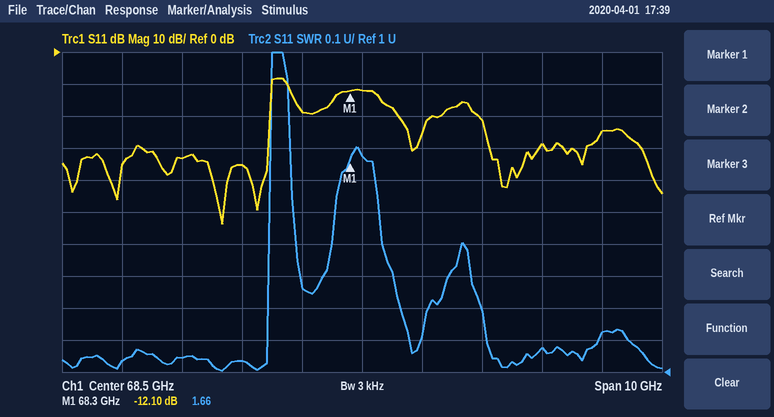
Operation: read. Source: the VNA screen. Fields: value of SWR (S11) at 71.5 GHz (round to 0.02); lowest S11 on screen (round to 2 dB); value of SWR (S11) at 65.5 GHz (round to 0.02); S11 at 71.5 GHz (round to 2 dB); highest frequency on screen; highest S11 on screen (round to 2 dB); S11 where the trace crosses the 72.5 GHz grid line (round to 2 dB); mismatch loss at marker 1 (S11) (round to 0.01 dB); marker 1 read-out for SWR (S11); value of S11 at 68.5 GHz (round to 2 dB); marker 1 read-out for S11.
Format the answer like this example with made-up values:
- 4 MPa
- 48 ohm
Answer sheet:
- 1.08
- -54 dB
- 1.04
- -28 dB
- 73.5 GHz
- -8 dB
- -24 dB
- 0.28 dB
- 1.66
- -12 dB
- -12.10 dB
